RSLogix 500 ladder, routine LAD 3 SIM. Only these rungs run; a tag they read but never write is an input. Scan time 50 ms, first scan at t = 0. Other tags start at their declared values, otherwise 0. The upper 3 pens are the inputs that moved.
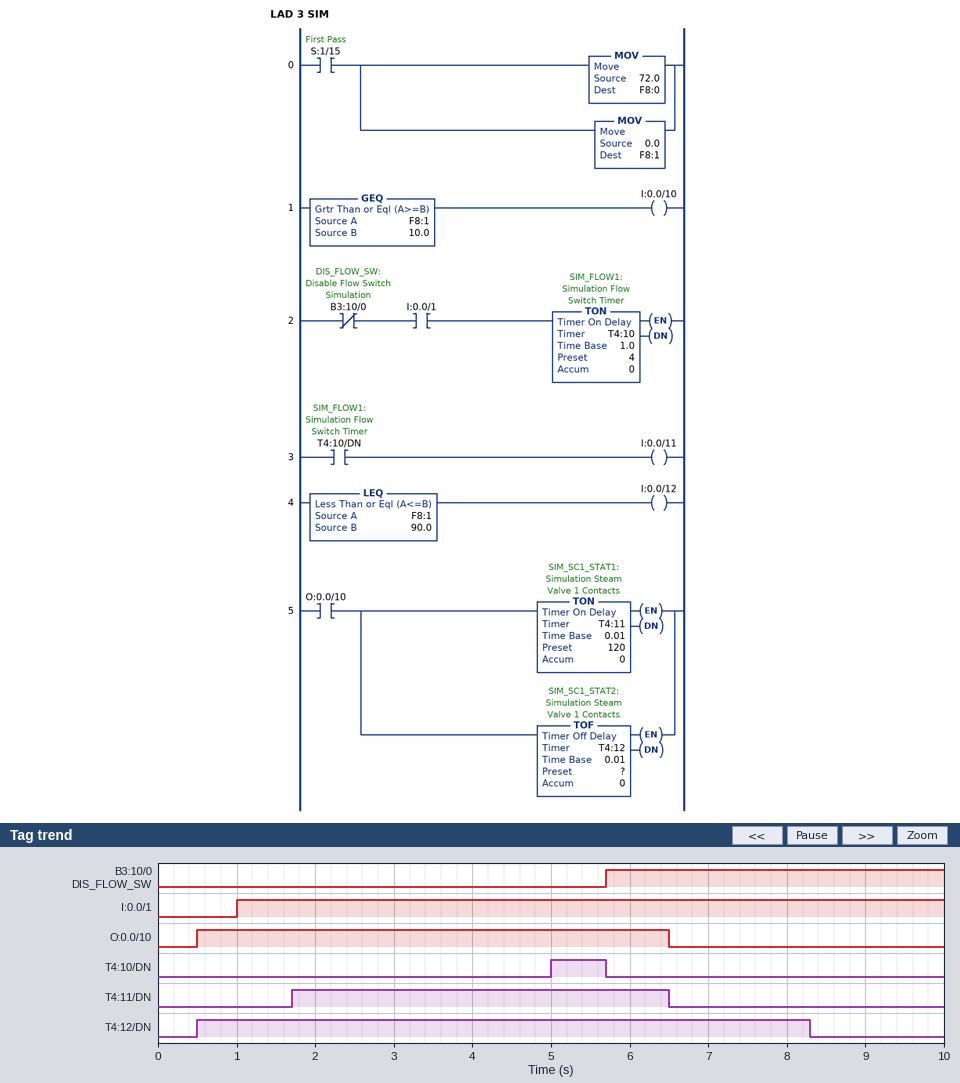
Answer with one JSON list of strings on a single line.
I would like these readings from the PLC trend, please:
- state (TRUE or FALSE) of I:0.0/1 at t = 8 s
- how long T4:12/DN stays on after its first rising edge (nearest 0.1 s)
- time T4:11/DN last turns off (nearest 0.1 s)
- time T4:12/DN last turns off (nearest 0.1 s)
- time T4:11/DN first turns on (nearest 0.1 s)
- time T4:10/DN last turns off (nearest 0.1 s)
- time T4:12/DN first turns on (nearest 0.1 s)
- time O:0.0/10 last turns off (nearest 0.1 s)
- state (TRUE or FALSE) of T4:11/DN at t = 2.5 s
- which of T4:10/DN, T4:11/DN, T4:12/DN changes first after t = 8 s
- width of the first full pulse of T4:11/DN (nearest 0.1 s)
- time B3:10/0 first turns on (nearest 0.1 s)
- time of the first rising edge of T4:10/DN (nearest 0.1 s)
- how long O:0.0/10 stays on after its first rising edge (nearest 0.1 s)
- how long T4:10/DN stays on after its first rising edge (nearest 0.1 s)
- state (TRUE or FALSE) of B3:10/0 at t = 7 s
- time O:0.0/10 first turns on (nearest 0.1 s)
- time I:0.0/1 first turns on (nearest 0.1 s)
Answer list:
["TRUE", "7.8 s", "6.5 s", "8.3 s", "1.7 s", "5.7 s", "0.5 s", "6.5 s", "TRUE", "T4:12/DN", "4.8 s", "5.7 s", "5.0 s", "6.0 s", "0.7 s", "TRUE", "0.5 s", "1.0 s"]
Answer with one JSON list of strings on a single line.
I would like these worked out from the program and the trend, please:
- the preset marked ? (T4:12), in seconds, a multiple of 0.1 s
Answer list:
["1.8 s"]
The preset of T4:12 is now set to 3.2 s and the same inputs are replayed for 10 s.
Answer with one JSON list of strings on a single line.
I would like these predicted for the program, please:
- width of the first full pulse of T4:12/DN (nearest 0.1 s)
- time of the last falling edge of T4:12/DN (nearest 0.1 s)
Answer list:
["9.2 s", "9.7 s"]
